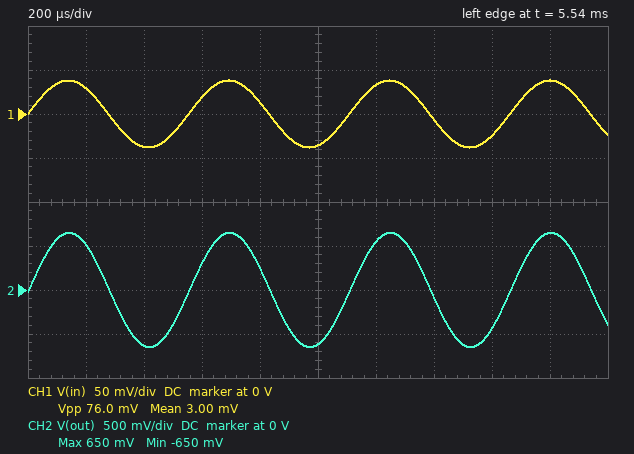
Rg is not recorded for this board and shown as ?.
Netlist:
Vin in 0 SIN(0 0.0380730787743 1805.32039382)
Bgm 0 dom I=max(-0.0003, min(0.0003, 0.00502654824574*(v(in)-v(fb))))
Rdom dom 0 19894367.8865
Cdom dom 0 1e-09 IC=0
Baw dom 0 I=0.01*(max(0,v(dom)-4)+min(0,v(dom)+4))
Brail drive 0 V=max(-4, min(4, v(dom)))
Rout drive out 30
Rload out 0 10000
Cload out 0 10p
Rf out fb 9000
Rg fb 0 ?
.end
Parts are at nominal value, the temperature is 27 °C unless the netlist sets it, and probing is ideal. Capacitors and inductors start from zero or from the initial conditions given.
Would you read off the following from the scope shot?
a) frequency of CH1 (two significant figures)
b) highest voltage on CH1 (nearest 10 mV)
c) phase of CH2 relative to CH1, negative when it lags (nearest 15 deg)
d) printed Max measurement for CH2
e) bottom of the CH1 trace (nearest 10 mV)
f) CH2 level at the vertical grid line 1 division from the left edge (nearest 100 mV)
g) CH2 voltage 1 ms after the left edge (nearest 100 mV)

1.8 kHz
40 mV
0 deg
650 mV
-40 mV
500 mV
-600 mV
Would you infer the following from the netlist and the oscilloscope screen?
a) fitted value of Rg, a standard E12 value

560 Ω
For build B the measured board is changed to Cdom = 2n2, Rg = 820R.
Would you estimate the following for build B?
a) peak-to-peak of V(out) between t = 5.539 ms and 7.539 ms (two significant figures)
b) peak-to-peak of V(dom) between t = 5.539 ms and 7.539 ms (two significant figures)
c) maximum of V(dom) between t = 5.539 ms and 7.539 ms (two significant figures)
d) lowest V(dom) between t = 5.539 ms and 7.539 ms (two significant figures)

910 mV
920 mV
460 mV
-460 mV
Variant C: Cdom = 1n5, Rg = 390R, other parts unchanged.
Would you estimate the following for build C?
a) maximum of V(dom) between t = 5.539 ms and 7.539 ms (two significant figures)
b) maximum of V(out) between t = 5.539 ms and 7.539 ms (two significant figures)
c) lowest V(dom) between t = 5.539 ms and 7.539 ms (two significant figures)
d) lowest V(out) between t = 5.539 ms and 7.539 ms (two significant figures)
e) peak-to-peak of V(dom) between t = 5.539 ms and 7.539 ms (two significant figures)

920 mV
910 mV
-920 mV
-910 mV
1.8 V
